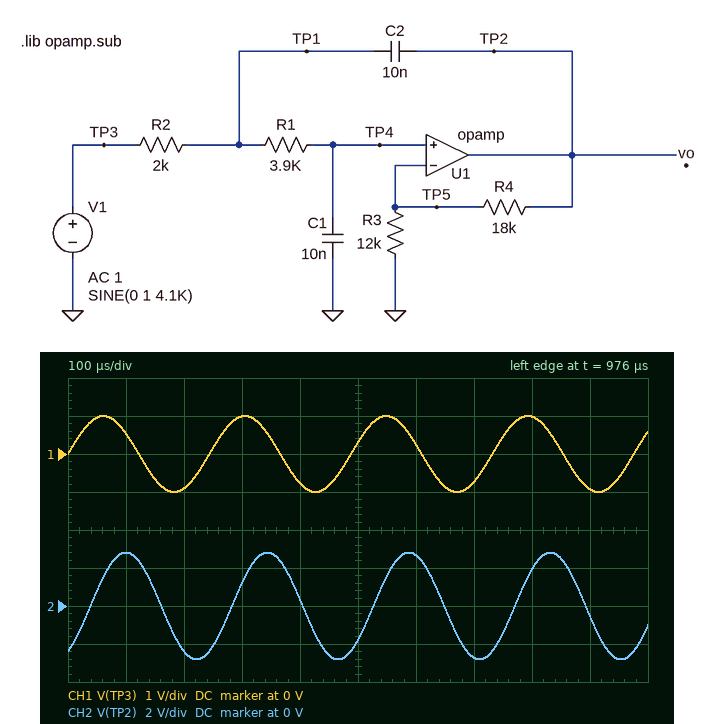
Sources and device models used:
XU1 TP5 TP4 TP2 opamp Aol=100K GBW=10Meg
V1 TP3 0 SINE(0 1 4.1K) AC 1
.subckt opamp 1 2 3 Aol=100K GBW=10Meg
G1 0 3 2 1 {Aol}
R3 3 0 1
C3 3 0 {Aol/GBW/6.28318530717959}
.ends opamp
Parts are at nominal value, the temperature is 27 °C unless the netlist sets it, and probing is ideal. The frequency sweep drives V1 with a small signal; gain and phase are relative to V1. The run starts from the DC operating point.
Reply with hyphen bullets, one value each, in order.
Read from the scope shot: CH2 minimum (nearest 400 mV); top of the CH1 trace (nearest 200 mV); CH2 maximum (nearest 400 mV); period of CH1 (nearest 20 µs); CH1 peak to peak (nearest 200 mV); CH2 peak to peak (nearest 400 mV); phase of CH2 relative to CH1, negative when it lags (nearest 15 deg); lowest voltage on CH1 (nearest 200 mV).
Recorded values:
- -2.8 V
- 1.0 V
- 2.8 V
- 240 µs
- 2.0 V
- 5.6 V
- -60 deg
- -1.0 V
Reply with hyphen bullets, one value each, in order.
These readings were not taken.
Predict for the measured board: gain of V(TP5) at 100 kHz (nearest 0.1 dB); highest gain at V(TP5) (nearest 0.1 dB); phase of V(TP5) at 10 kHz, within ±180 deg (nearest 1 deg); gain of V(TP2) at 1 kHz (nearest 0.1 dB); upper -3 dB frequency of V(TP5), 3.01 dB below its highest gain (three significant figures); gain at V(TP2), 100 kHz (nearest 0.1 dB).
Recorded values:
- -49.8 dB
- 1.0 dB
- -139 deg
- 8.1 dB
- 6.61 kHz
- -41.8 dB
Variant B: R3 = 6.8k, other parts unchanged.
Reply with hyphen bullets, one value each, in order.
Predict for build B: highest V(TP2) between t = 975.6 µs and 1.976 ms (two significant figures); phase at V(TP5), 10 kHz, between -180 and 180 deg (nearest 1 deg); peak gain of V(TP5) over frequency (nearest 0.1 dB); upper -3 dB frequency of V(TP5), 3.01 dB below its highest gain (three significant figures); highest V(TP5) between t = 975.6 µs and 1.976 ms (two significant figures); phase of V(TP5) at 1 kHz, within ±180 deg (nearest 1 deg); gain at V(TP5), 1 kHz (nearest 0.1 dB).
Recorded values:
- 7.3 V
- -170 deg
- 13.3 dB
- 6.20 kHz
- 2.0 V
- -2 deg
- 0.3 dB
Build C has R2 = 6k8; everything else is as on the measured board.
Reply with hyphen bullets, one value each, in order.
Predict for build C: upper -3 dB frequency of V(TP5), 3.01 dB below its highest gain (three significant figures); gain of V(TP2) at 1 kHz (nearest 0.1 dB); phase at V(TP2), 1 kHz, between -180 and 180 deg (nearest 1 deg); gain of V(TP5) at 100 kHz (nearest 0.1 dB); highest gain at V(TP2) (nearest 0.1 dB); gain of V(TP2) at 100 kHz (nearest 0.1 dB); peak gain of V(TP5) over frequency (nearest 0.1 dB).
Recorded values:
- 3.23 kHz
- 8.9 dB
- -2 deg
- -60.4 dB
- 28.2 dB
- -52.5 dB
- 20.3 dB
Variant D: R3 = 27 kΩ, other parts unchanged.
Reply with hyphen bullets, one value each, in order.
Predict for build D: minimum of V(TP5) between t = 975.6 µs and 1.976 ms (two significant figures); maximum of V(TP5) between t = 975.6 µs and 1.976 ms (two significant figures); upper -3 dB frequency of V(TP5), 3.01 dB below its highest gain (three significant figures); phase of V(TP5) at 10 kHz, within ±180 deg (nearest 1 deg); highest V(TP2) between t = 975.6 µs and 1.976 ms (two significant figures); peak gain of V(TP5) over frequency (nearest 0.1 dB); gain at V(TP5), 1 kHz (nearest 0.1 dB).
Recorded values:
- -790 mV
- 790 mV
- 4.83 kHz
- -126 deg
- 1.3 V
- 0 dB
- -0.1 dB
